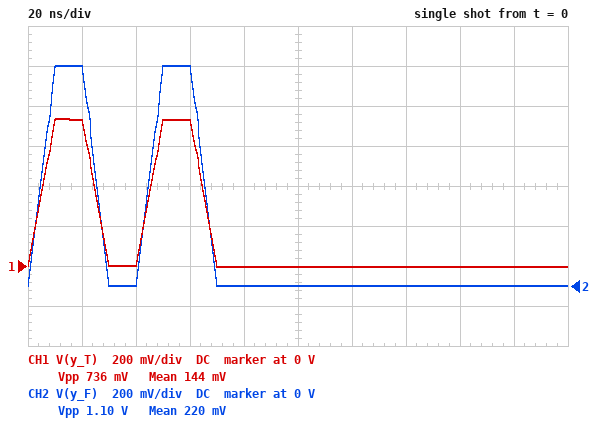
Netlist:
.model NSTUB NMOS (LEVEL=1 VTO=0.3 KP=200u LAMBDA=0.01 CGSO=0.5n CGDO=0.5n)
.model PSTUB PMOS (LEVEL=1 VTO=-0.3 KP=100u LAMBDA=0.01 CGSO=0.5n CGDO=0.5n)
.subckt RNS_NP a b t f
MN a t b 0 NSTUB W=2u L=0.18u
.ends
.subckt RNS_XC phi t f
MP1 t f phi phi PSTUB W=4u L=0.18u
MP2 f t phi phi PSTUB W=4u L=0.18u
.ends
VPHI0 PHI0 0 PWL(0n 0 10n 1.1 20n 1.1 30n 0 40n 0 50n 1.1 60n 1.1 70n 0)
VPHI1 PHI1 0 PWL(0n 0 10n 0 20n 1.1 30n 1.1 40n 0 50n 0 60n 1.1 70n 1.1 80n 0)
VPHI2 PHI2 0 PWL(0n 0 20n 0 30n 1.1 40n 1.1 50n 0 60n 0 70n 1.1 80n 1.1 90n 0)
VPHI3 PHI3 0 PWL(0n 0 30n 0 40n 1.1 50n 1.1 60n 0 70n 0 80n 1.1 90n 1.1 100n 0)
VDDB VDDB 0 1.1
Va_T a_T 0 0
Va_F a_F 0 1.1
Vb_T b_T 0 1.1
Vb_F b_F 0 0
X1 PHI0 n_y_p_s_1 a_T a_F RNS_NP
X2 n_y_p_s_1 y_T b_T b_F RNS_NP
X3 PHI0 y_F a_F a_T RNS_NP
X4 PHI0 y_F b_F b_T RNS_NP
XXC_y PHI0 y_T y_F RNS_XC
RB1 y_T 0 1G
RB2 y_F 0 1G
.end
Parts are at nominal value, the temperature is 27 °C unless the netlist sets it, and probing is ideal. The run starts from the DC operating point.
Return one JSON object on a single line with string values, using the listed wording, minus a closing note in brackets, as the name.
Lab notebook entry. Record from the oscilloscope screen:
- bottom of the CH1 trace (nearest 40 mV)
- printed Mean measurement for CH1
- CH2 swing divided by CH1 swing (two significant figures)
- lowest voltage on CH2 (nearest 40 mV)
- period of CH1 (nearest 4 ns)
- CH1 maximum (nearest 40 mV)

{"bottom of the CH1 trace": "0 V", "printed Mean measurement for CH1": "144 mV", "CH2 swing divided by CH1 swing": "1.5", "lowest voltage on CH2": "0 V", "period of CH1": "40 ns", "CH1 maximum": "720 mV"}
